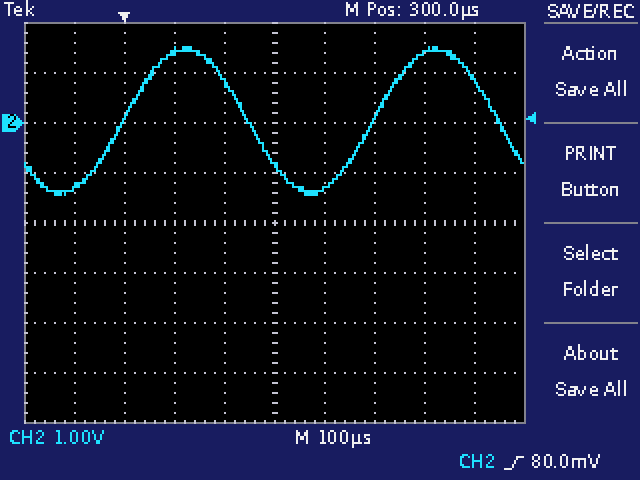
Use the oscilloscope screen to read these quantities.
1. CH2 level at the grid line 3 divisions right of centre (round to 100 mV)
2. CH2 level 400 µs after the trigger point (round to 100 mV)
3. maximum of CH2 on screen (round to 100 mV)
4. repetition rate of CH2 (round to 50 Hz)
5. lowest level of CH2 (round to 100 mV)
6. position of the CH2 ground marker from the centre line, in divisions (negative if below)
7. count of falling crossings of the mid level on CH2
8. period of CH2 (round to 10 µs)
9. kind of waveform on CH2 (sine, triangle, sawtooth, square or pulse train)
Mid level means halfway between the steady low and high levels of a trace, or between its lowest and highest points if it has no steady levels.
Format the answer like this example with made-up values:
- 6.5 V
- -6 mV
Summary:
- 1.4 V
- -1.3 V
- 1.5 V
- 2.00 kHz
- -1.4 V
- +2.0 div
- 2
- 500 µs
- sine
